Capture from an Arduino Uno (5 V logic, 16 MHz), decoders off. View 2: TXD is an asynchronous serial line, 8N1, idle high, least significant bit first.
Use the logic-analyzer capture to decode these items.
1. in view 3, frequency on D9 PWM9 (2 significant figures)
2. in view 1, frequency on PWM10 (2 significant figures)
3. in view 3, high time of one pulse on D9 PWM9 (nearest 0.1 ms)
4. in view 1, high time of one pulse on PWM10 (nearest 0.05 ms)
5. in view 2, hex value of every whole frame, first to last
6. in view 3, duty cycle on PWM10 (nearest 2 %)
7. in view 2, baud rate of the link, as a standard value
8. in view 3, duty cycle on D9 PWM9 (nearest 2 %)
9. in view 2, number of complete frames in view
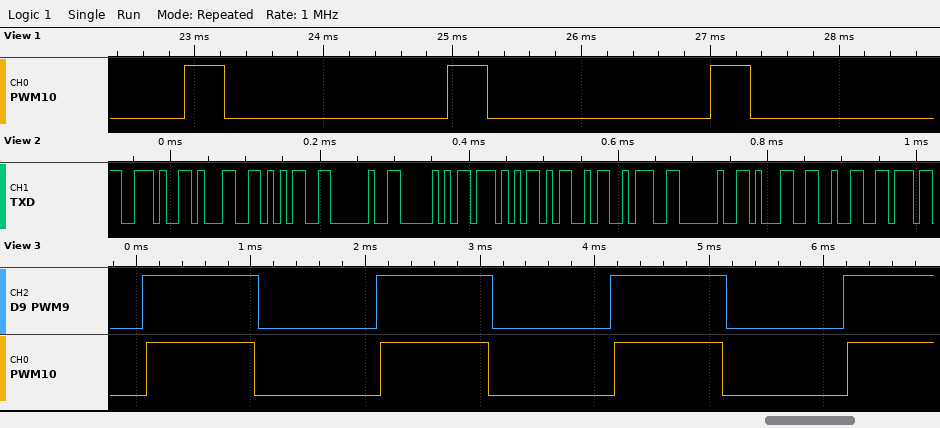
490 Hz
490 Hz
1.0 ms
0.30 ms
2E 31 35 20 50 57 4D 3A 20 31 32
46 %
115200 baud
50 %
11
